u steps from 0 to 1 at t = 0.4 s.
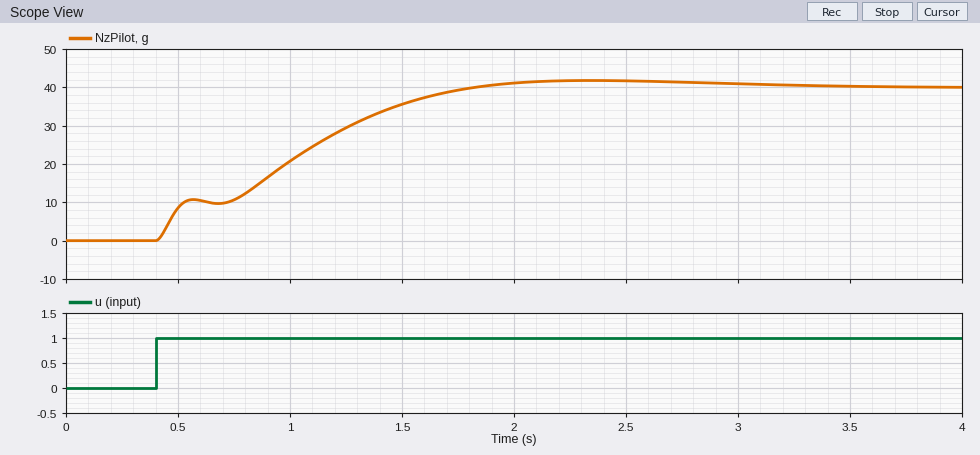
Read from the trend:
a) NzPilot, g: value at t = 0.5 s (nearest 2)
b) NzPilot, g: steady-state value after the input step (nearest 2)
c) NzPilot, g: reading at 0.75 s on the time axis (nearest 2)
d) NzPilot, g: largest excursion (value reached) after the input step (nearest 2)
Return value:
8
40
10
42
